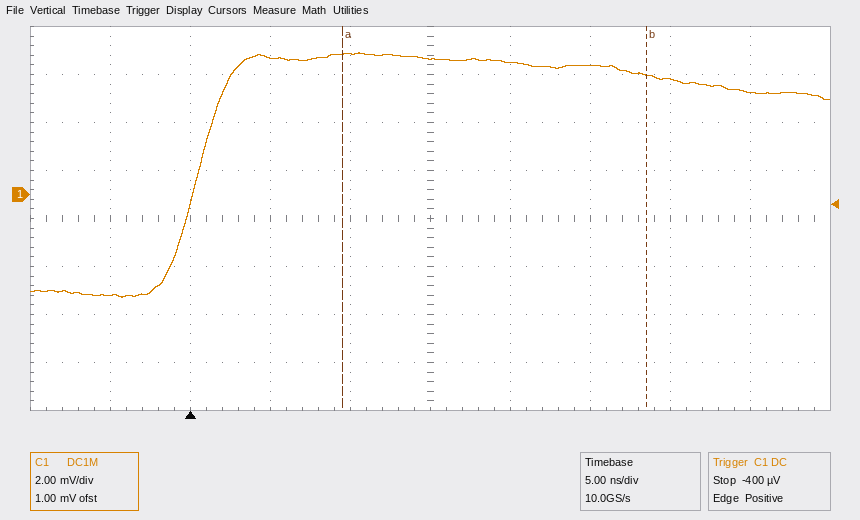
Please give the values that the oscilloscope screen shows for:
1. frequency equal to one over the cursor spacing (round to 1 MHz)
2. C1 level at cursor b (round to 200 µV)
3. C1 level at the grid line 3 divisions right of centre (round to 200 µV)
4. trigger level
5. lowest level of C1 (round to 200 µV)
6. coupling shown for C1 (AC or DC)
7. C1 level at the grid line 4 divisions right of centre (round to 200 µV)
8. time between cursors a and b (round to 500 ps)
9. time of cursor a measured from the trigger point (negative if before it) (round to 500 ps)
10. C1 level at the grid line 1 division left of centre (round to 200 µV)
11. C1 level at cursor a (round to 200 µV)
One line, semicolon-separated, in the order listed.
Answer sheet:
53 MHz; 5.0 mV; 4.8 mV; -400 µV; -4.2 mV; DC; 4.2 mV; 19.0 ns; +9.5 ns; 5.8 mV; 5.8 mV
